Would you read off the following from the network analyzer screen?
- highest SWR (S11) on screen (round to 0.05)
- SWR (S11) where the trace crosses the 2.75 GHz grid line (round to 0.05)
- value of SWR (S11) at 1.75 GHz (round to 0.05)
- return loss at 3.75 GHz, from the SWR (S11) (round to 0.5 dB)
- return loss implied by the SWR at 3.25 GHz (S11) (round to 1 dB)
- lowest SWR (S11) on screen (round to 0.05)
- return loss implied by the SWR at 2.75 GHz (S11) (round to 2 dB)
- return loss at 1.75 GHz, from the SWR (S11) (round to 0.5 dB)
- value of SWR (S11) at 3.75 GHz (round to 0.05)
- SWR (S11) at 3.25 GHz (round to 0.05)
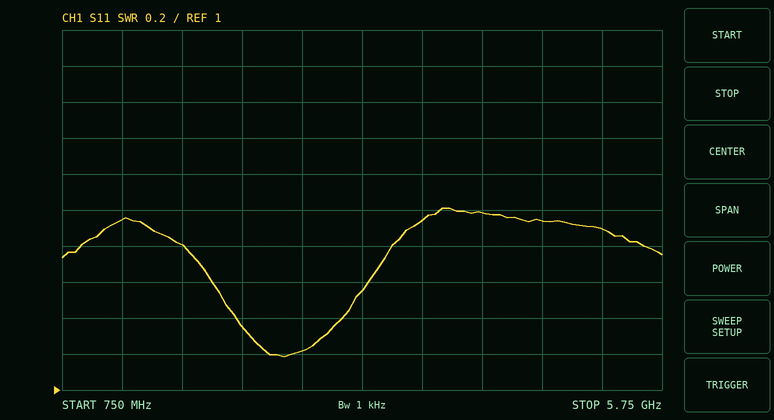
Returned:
2.00
1.20
1.80
10.0 dB
13 dB
1.20
20 dB
11.0 dB
1.95
1.55
